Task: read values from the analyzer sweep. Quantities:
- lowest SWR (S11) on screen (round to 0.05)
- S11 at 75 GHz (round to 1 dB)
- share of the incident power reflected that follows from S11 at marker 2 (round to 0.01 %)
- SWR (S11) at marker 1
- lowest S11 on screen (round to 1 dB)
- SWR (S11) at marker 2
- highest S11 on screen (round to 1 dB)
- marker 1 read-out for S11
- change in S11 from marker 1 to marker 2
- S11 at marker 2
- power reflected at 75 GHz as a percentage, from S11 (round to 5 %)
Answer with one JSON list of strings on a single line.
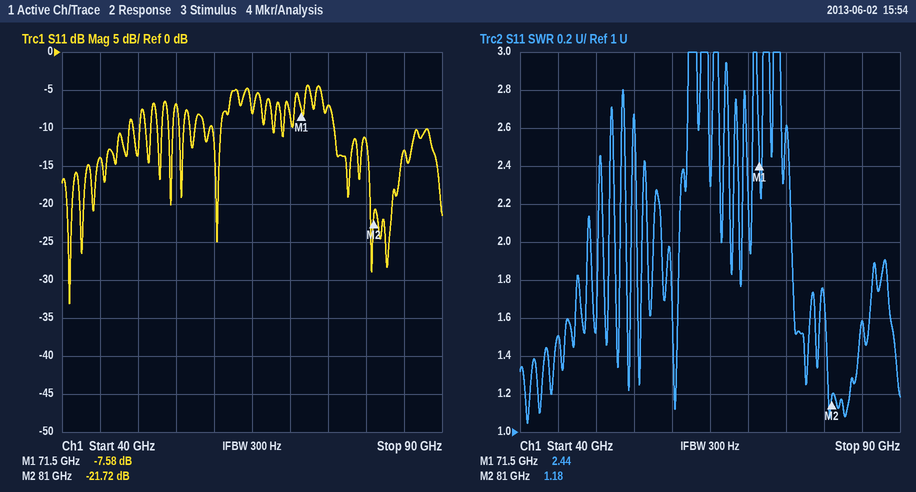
["1.05", "-7 dB", "0.67 %", "2.44", "-33 dB", "1.18", "-4 dB", "-7.58 dB", "-14.14 dB", "-21.72 dB", "20 %"]
